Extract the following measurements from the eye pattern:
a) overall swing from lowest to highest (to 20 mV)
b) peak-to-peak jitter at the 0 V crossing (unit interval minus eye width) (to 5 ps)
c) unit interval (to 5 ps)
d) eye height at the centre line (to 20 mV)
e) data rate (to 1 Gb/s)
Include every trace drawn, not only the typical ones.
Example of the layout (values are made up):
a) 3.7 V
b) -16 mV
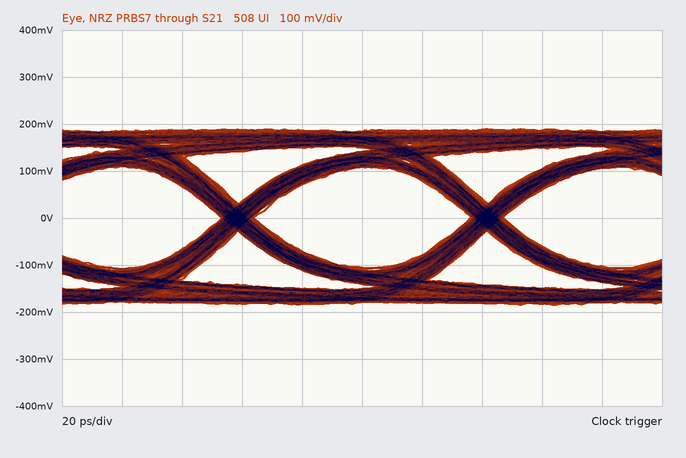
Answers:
a) 380 mV
b) 10 ps
c) 85 ps
d) 220 mV
e) 12 Gb/s
